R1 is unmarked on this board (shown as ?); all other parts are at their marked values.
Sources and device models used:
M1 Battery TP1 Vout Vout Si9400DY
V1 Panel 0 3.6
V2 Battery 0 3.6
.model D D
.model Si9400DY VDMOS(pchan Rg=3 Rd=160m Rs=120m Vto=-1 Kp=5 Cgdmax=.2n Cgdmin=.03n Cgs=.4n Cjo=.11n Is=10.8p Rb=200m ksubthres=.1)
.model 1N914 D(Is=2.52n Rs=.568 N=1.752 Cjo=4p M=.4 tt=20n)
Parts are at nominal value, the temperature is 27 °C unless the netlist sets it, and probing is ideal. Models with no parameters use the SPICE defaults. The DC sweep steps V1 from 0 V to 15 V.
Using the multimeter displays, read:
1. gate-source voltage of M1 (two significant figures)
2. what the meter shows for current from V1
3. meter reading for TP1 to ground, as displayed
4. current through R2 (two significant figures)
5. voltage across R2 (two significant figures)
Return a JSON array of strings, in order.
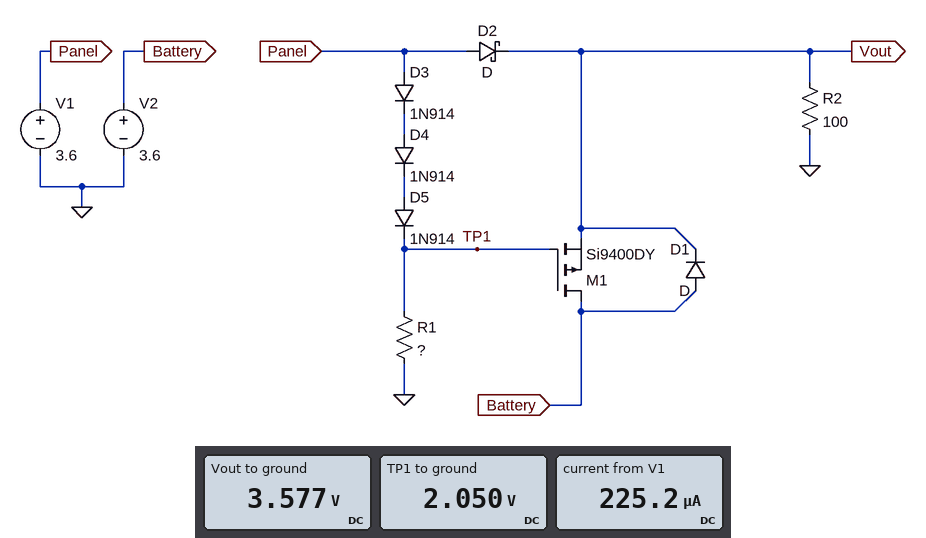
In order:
["-1.5 V", "225.2 µA", "2.050 V", "36 mA", "3.6 V"]
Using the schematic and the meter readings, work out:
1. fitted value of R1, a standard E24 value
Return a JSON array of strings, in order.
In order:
["9.1 kΩ"]
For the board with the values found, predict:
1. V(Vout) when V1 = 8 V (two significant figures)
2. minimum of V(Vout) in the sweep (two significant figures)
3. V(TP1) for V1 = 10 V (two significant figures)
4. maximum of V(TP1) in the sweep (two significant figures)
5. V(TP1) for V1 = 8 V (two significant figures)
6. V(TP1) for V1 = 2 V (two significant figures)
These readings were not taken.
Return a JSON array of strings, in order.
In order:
["7.2 V", "3.4 V", "8.3 V", "13 V", "6.3 V", "610 mV"]
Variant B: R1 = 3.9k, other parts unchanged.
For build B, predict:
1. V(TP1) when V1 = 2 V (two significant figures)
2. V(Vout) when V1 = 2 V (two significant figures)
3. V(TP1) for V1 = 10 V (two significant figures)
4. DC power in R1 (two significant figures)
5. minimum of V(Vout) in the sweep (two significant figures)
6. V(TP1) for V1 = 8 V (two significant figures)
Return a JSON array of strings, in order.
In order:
["520 mV", "3.6 V", "8.1 V", "970 µW", "3.5 V", "6.2 V"]
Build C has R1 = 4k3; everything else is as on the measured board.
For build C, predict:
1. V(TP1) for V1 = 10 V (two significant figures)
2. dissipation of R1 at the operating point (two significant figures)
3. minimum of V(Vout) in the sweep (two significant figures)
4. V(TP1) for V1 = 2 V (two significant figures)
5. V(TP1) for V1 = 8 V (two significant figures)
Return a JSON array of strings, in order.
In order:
["8.2 V", "890 µW", "3.5 V", "530 mV", "6.2 V"]
